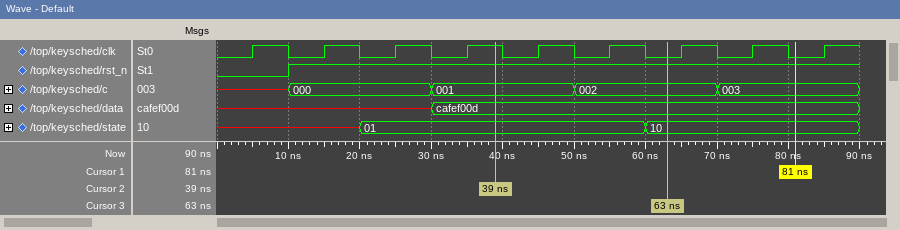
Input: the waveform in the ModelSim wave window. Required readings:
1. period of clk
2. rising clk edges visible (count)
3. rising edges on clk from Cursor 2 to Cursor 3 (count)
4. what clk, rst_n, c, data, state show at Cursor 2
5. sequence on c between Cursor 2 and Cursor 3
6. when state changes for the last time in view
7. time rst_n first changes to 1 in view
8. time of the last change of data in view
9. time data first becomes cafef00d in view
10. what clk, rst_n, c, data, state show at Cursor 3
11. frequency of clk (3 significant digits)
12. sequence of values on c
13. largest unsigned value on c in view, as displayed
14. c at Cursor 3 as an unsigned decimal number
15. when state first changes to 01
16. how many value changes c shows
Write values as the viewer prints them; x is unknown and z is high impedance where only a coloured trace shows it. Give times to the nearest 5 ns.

10 ns
9
2
clk=1, rst_n=1, c=001, data=cafef00d, state=01
001, 002
60 ns
10 ns
30 ns
30 ns
clk=0, rst_n=1, c=002, data=cafef00d, state=10
100 MHz
x, 000, 001, 002, 003
003
2
20 ns
4
